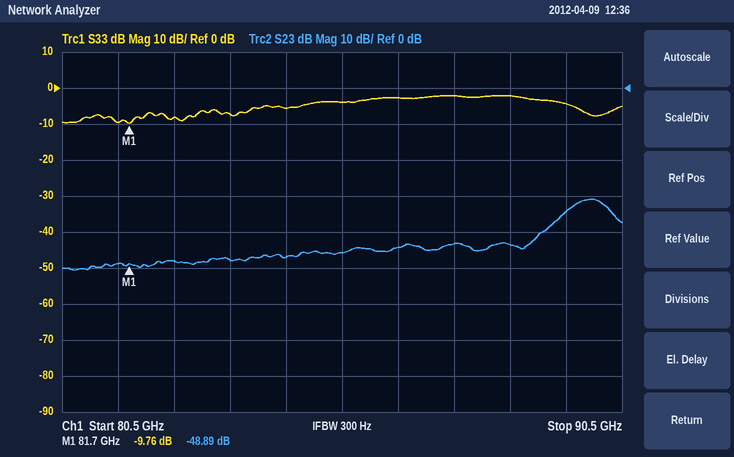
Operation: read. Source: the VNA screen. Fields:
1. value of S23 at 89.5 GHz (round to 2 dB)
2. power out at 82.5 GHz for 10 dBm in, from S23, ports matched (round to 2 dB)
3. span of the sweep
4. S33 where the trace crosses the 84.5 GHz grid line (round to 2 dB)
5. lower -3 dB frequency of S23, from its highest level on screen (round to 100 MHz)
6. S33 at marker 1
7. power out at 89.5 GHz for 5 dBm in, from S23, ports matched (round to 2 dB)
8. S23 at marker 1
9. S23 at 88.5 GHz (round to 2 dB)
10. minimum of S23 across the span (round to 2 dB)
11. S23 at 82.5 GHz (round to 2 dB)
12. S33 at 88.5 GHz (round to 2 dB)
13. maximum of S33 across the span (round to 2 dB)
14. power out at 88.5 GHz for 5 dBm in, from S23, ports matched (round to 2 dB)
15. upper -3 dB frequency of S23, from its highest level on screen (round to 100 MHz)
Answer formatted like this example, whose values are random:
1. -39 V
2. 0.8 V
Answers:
1. -34 dB
2. -38 dBm
3. 10 GHz
4. -6 dB
5. 89.5 GHz
6. -9.76 dB
7. -30 dBm
8. -48.89 dB
9. -44 dB
10. -50 dB
11. -48 dB
12. -2 dB
13. -2 dB
14. -38 dBm
15. 90.3 GHz
